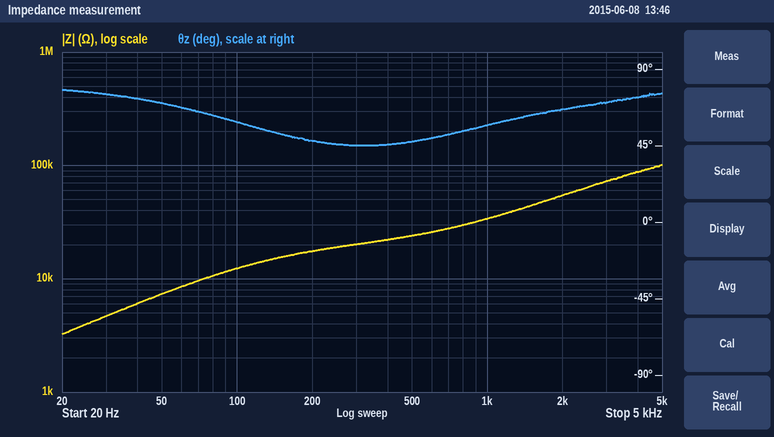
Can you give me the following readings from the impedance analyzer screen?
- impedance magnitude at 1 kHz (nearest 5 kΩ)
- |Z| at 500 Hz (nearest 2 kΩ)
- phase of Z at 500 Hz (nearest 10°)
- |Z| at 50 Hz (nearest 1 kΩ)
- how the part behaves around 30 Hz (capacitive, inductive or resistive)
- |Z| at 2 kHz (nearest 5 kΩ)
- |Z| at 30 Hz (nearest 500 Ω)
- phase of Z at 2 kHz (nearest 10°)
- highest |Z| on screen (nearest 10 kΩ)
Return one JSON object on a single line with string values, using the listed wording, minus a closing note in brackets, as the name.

{"impedance magnitude at 1 kHz": "35 kΩ", "|Z| at 500 Hz": "24 kΩ", "phase of Z at 500 Hz": "50°", "|Z| at 50 Hz": "7 kΩ", "how the part behaves around 30 Hz": "inductive", "|Z| at 2 kHz": "55 kΩ", "|Z| at 30 Hz": "4.5 kΩ", "phase of Z at 2 kHz": "70°", "highest |Z| on screen": "100 kΩ"}
